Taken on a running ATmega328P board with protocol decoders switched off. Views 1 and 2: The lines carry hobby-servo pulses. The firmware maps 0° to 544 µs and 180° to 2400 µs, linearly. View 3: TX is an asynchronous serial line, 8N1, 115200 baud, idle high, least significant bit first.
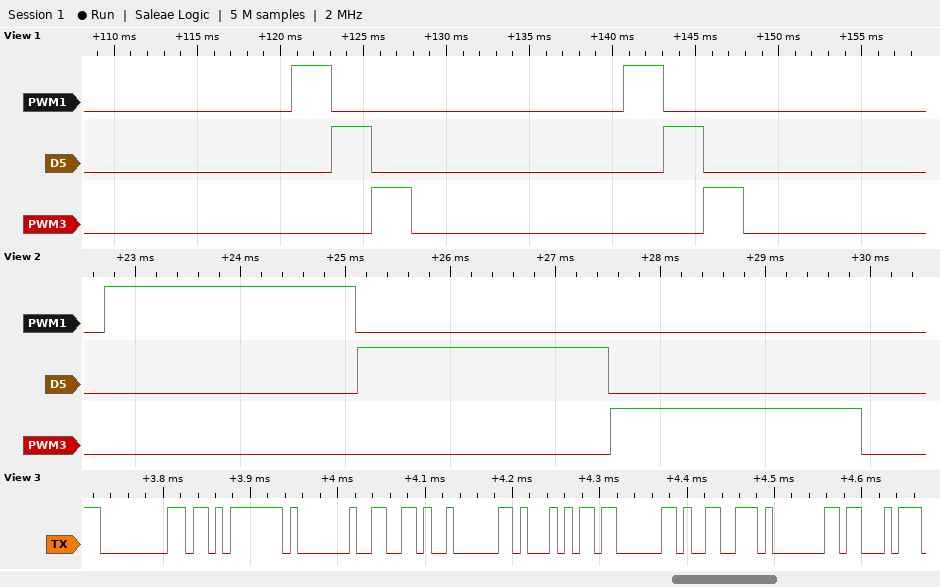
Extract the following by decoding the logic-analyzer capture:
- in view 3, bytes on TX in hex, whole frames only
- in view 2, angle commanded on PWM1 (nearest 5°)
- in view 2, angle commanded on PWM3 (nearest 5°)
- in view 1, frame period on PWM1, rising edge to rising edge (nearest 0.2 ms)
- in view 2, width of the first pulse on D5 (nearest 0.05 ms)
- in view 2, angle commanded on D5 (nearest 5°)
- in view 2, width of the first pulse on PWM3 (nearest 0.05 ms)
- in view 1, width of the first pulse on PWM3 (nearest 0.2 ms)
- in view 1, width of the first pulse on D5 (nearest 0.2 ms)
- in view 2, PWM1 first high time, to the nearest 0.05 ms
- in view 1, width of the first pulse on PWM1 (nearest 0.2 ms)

0x00 0xEB 0x01 0x66 0x02 0x51 0x03 0x99 0x01 0xA3
180°
180°
20.0 ms
2.40 ms
180°
2.40 ms
2.4 ms
2.4 ms
2.40 ms
2.4 ms
